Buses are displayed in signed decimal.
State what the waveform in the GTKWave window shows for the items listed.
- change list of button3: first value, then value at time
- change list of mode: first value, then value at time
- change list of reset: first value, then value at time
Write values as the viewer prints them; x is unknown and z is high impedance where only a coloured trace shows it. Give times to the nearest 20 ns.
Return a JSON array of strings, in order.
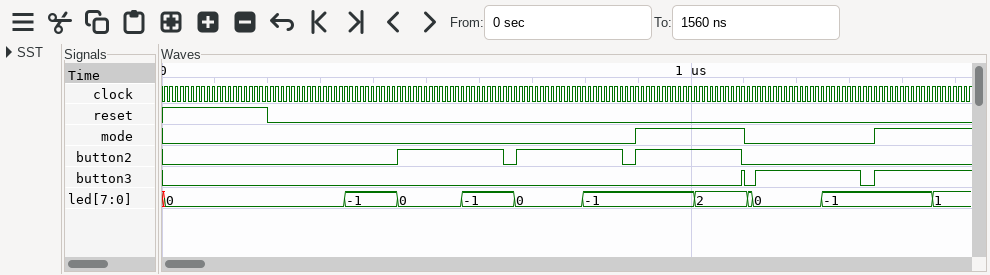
["0, 1 at 1100 ns, 0 at 1100 ns, 1 at 1120 ns, 0 at 1320 ns, 1 at 1340 ns", "0, 1 at 900 ns, 0 at 1100 ns, 1 at 1340 ns", "1, 0 at 200 ns"]
